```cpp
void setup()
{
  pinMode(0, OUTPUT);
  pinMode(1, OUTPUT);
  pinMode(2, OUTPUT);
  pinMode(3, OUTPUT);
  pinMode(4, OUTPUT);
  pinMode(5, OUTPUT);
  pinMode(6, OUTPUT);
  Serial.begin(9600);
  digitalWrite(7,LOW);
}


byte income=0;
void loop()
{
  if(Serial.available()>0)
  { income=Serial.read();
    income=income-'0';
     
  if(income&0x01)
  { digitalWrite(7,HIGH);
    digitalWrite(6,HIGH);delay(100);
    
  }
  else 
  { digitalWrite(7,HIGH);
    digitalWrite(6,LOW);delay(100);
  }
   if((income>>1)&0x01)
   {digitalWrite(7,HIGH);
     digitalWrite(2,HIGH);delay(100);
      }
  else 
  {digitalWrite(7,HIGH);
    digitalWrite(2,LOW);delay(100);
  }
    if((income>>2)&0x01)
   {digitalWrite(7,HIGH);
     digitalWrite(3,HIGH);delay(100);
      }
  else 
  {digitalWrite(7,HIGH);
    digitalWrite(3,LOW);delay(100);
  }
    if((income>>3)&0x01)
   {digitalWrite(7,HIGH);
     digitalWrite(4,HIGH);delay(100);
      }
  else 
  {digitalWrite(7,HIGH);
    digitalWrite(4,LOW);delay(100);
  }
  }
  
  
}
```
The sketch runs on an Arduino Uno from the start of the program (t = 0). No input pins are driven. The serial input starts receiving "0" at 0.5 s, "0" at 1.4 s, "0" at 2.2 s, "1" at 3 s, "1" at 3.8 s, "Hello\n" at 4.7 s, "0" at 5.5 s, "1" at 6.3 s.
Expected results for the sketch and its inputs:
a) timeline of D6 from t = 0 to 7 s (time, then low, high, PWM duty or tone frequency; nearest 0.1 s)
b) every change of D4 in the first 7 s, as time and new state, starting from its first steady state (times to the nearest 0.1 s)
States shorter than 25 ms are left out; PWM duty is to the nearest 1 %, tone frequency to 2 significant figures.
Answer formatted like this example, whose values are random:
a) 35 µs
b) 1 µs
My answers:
a) 0 s low; 3 s high; 4.7 s low; 5.1 s high; 5.5 s low; 6.3 s high; 6.7 s low
b) 0 s low; 5 s high; 5.4 s low; 5.8 s high
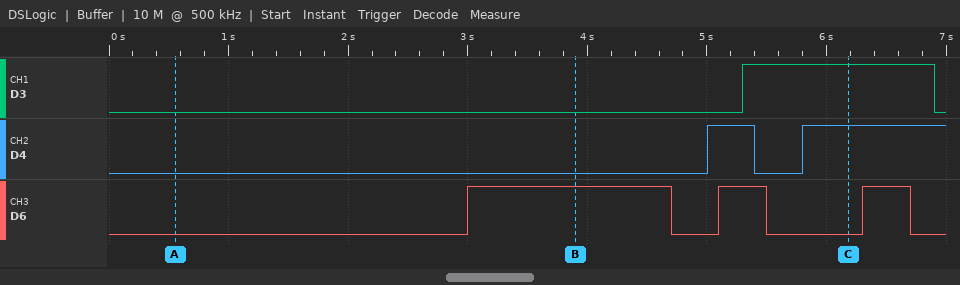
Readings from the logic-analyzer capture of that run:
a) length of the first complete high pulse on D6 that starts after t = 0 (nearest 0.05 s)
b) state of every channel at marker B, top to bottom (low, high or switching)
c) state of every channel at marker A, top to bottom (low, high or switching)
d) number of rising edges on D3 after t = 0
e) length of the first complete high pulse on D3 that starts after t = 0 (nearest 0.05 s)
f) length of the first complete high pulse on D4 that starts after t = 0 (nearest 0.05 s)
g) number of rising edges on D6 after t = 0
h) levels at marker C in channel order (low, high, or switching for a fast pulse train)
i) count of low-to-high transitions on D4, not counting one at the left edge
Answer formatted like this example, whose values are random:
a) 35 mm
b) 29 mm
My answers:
a) 1.70 s
b) D3 low, D4 low, D6 high
c) D3 low, D4 low, D6 low
d) 1
e) 1.60 s
f) 0.40 s
g) 3
h) D3 high, D4 high, D6 low
i) 2
